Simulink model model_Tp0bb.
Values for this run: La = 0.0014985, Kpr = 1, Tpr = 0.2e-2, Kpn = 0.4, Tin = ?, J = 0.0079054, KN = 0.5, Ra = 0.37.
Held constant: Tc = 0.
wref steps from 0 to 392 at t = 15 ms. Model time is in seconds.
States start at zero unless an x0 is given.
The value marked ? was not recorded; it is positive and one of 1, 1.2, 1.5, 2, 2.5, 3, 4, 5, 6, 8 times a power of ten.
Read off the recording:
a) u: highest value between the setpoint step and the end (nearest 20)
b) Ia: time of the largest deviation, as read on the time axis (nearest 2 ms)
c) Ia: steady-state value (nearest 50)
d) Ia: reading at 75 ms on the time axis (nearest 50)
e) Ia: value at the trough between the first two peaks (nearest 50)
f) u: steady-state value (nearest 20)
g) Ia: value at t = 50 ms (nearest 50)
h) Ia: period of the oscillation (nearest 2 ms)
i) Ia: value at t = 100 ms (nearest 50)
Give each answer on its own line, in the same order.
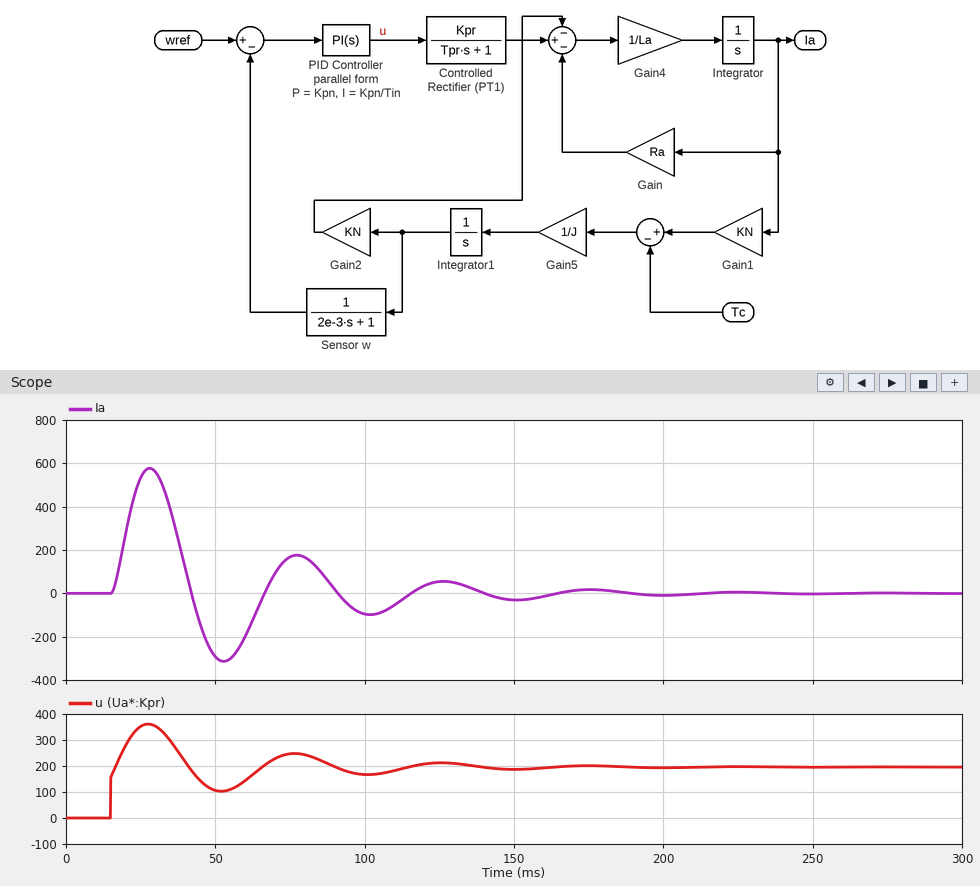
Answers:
360
28 ms
0
150
-300
200
-300
50 ms
-100
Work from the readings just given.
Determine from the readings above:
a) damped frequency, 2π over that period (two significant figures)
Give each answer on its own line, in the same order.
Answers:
0.13 rad/ms
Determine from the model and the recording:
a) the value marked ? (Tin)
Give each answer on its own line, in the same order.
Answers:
0.006
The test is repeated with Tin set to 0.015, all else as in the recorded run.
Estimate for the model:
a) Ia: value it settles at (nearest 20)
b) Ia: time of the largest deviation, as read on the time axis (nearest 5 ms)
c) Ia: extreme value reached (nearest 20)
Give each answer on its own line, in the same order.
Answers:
0
25 ms
380
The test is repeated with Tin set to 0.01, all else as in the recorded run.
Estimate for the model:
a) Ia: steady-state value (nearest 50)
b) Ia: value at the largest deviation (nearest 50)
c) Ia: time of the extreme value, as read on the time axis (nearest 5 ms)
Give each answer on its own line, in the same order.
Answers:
0
450
25 ms
